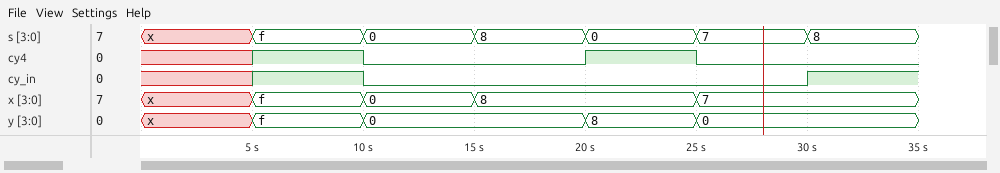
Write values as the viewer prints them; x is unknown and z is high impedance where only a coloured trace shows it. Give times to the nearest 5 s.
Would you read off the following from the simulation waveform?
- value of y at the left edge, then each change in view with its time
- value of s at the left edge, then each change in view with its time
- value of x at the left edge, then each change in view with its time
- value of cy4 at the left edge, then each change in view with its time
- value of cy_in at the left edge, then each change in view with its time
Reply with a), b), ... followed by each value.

a) x, f at 5 s, 0 at 10 s, 8 at 20 s, 0 at 25 s
b) x, f at 5 s, 0 at 10 s, 8 at 15 s, 0 at 20 s, 7 at 25 s, 8 at 30 s
c) x, f at 5 s, 0 at 10 s, 8 at 15 s, 7 at 25 s
d) x, 1 at 5 s, 0 at 10 s, 1 at 20 s, 0 at 25 s
e) x, 1 at 5 s, 0 at 10 s, 1 at 30 s
